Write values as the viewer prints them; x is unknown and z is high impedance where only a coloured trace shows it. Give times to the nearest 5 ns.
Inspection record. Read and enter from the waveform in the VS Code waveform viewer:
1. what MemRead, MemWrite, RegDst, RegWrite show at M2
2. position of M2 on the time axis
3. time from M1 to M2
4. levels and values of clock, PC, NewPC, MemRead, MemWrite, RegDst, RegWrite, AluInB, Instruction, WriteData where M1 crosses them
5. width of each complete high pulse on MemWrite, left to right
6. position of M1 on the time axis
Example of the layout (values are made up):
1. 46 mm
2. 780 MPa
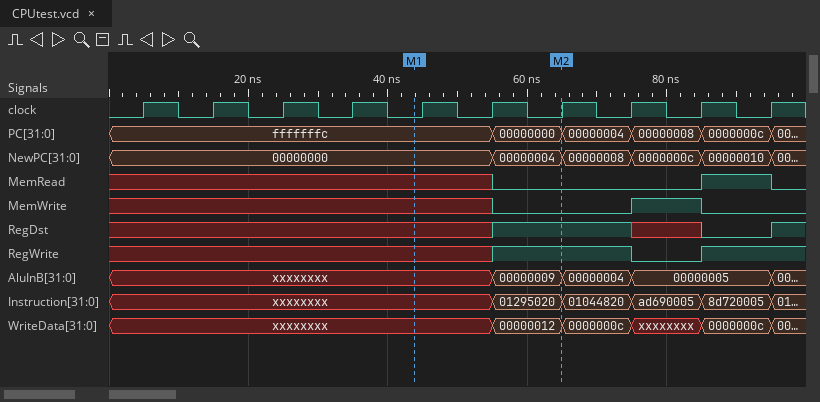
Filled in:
1. MemRead=0, MemWrite=0, RegDst=1, RegWrite=1
2. 65 ns
3. 20 ns
4. clock=0, PC=fffffffc, NewPC=00000000, MemRead=x, MemWrite=x, RegDst=x, RegWrite=x, AluInB=xxxxxxxx, Instruction=xxxxxxxx, WriteData=xxxxxxxx
5. 10 ns
6. 45 ns
